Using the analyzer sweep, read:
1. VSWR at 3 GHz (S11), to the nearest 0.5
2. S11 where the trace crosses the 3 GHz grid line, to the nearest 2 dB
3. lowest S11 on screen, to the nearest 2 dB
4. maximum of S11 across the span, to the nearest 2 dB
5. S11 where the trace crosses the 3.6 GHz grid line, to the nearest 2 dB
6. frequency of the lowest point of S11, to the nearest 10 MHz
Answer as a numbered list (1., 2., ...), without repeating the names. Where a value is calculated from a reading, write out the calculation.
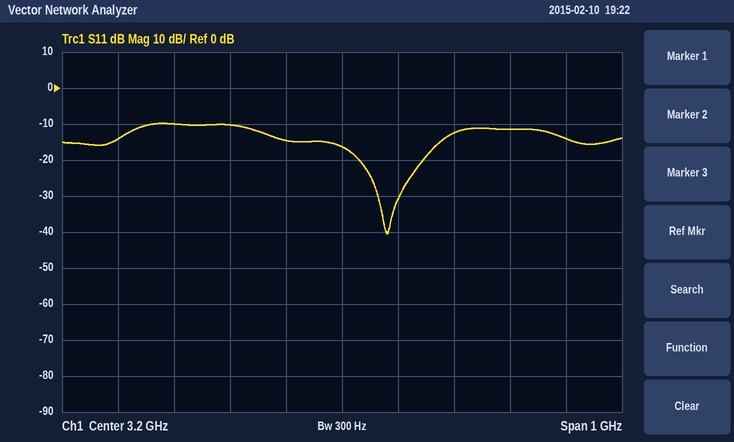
1. |Γ| = 10^(-10/20) = 0.3162; VSWR = (1 + 0.3162)/(1 − 0.3162) ≈ 1.92, so 2.0 to the nearest 0.5
2. -10 dB
3. -40 dB
4. -10 dB
5. -14 dB
6. 3.28 GHz
